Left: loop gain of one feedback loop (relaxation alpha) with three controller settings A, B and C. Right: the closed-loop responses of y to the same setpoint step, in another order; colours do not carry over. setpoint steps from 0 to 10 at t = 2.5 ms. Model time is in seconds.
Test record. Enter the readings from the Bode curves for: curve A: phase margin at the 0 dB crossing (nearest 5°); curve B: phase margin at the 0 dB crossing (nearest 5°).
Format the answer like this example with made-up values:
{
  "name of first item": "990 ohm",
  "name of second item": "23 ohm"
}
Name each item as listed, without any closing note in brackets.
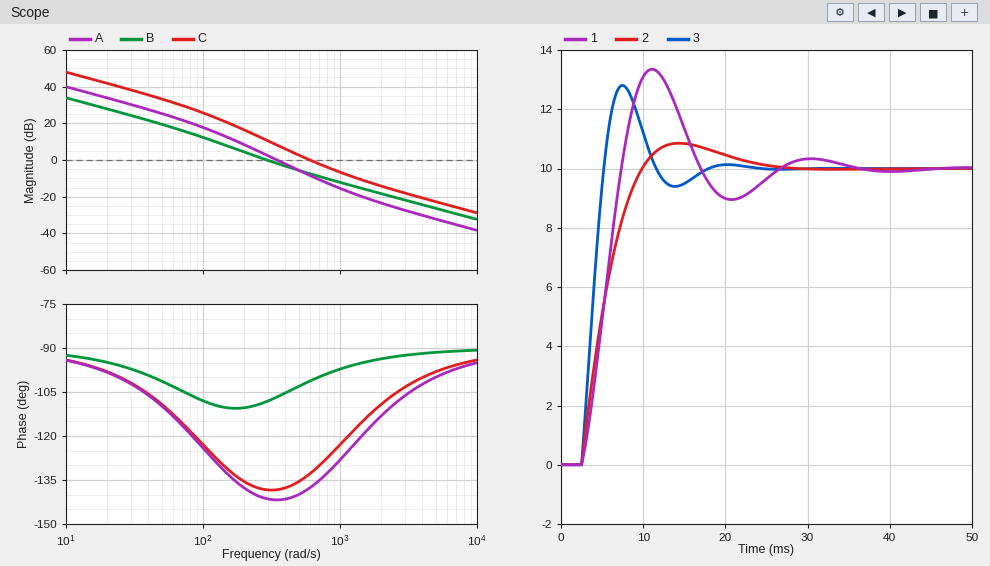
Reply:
{
  "curve A: phase margin at the 0 dB crossing": "40°",
  "curve B: phase margin at the 0 dB crossing": "70°"
}
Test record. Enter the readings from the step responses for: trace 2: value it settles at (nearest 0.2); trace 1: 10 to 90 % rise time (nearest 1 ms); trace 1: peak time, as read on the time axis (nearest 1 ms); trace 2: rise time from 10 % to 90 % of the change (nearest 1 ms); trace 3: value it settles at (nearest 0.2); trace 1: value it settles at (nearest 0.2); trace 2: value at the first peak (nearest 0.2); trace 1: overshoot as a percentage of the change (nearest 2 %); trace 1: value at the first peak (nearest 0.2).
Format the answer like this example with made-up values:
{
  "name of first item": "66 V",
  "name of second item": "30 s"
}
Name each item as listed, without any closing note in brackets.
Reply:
{
  "trace 2: value it settles at": "10.0",
  "trace 1: 10 to 90 % rise time": "4 ms",
  "trace 1: peak time, as read on the time axis": "11 ms",
  "trace 2: rise time from 10 % to 90 % of the change": "5 ms",
  "trace 3: value it settles at": "10.0",
  "trace 1: value it settles at": "10.0",
  "trace 2: value at the first peak": "10.8",
  "trace 1: overshoot as a percentage of the change": "34 %",
  "trace 1: value at the first peak": "13.4"
}
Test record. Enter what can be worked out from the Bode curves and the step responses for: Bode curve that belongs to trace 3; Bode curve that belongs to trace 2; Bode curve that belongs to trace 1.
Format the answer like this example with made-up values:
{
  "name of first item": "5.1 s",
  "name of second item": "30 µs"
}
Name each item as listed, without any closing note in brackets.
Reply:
{
  "Bode curve that belongs to trace 3": "C",
  "Bode curve that belongs to trace 2": "B",
  "Bode curve that belongs to trace 1": "A"
}
